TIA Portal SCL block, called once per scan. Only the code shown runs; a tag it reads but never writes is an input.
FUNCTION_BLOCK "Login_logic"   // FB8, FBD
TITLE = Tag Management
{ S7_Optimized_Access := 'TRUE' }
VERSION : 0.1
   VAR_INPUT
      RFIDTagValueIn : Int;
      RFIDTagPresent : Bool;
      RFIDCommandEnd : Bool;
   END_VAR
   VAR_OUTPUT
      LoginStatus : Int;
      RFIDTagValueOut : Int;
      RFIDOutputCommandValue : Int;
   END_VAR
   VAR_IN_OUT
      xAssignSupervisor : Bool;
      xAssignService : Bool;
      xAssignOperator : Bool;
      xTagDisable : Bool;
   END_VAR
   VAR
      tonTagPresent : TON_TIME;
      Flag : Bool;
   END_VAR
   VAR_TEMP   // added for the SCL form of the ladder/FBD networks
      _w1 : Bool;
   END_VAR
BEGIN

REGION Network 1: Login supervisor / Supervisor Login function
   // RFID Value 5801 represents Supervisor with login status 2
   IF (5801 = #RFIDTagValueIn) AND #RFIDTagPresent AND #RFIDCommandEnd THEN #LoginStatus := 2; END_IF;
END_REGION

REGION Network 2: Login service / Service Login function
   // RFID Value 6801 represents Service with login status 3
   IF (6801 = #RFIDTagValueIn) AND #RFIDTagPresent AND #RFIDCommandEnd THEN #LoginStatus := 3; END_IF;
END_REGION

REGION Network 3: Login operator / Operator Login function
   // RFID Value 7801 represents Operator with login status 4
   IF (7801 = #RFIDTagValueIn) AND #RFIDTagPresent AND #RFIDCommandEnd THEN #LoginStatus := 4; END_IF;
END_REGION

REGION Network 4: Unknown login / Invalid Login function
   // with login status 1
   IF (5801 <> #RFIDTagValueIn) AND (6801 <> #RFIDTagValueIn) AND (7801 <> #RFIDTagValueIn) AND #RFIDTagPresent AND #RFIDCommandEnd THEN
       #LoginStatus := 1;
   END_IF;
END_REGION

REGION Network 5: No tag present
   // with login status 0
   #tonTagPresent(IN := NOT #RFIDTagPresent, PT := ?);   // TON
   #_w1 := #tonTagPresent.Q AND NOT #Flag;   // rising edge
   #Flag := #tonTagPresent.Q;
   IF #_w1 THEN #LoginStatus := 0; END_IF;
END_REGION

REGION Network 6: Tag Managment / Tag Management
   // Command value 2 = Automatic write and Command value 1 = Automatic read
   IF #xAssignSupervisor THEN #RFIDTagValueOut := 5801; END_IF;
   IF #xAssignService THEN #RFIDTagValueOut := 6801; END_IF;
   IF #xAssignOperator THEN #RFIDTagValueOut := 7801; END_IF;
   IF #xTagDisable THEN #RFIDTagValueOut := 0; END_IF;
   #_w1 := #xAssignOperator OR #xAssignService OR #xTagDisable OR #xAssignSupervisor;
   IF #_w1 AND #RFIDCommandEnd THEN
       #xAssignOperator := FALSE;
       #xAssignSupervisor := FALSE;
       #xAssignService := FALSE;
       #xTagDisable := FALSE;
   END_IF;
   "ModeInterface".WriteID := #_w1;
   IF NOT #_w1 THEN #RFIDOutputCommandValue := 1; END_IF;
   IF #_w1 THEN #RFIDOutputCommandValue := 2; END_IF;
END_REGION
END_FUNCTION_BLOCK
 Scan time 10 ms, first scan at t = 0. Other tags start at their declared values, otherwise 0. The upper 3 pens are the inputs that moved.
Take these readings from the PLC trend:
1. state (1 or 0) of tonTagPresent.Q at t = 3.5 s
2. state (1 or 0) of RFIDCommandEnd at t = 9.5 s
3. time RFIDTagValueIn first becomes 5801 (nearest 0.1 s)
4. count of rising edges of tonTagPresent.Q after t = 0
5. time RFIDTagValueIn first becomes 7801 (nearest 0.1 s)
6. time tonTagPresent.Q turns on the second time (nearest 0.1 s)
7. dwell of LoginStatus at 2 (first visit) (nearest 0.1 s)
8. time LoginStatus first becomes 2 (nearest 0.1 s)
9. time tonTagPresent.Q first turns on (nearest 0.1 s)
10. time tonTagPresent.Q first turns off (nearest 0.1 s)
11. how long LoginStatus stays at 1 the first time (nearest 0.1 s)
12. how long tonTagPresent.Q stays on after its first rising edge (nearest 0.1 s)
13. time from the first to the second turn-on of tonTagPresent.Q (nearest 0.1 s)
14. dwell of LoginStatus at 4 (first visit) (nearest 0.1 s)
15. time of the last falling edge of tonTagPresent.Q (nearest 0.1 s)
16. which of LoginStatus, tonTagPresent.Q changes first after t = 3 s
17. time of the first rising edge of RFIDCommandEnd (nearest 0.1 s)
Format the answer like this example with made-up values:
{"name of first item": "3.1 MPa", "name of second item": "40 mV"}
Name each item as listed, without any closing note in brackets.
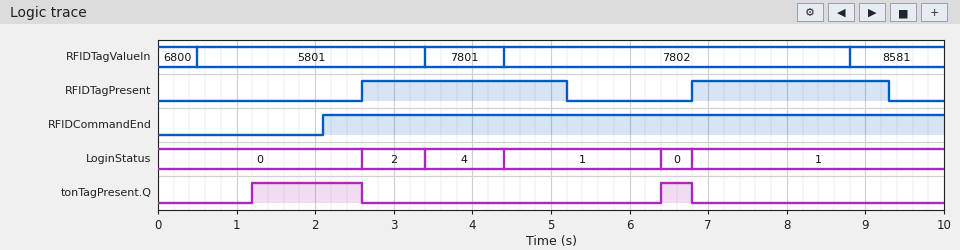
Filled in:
{"state (1 or 0) of tonTagPresent.Q at t = 3.5 s": "0", "state (1 or 0) of RFIDCommandEnd at t = 9.5 s": "1", "time RFIDTagValueIn first becomes 5801": "0.5 s", "count of rising edges of tonTagPresent.Q after t = 0": "2", "time RFIDTagValueIn first becomes 7801": "3.4 s", "time tonTagPresent.Q turns on the second time": "6.4 s", "dwell of LoginStatus at 2 (first visit)": "0.8 s", "time LoginStatus first becomes 2": "2.6 s", "time tonTagPresent.Q first turns on": "1.2 s", "time tonTagPresent.Q first turns off": "2.6 s", "how long LoginStatus stays at 1 the first time": "2.0 s", "how long tonTagPresent.Q stays on after its first rising edge": "1.4 s", "time from the first to the second turn-on of tonTagPresent.Q": "5.2 s", "dwell of LoginStatus at 4 (first visit)": "1.0 s", "time of the last falling edge of tonTagPresent.Q": "6.8 s", "which of LoginStatus, tonTagPresent.Q changes first after t = 3 s": "LoginStatus", "time of the first rising edge of RFIDCommandEnd": "2.1 s"}
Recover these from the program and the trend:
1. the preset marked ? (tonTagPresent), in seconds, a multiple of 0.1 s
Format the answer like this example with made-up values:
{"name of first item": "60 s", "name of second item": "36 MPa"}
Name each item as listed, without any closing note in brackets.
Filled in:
{"the preset marked ? (tonTagPresent), in seconds, a multiple of 0.1 s": "1.2 s"}
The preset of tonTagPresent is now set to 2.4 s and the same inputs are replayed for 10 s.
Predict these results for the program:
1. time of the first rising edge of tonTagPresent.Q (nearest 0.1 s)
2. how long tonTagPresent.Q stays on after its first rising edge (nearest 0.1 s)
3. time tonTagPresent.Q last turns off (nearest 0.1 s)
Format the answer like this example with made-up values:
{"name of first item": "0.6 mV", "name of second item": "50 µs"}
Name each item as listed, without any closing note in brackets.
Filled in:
{"time of the first rising edge of tonTagPresent.Q": "2.4 s", "how long tonTagPresent.Q stays on after its first rising edge": "0.2 s", "time tonTagPresent.Q last turns off": "2.6 s"}
